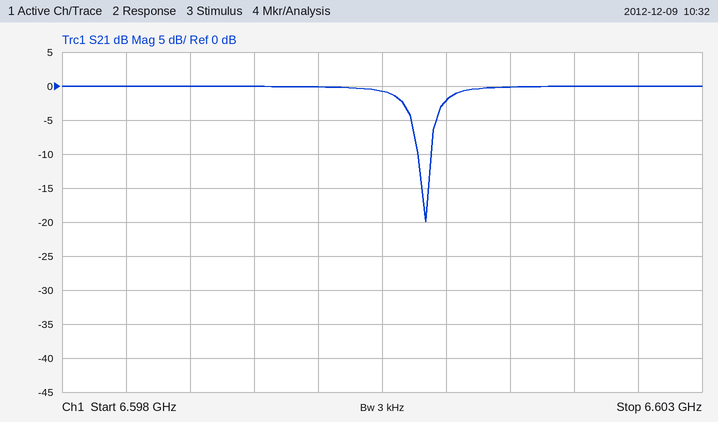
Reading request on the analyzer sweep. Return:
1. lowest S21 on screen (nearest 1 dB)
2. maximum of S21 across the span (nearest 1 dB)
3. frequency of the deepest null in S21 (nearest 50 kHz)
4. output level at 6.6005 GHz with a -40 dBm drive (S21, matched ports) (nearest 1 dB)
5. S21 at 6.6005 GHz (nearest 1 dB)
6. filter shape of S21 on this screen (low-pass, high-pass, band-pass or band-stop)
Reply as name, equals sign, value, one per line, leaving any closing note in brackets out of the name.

lowest S21 on screen = -20 dB
maximum of S21 across the span = 0 dB
frequency of the deepest null in S21 = 6.60085 GHz
output level at 6.6005 GHz with a -40 dBm drive (S21, matched ports) = -41 dBm
S21 at 6.6005 GHz = -1 dB
filter shape of S21 on this screen = band-stop
